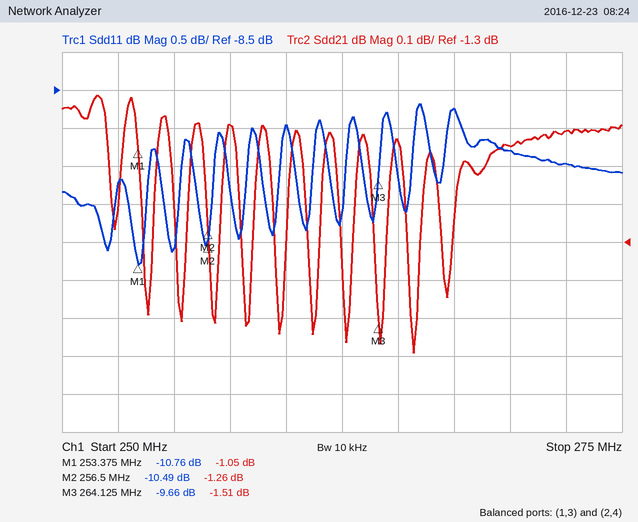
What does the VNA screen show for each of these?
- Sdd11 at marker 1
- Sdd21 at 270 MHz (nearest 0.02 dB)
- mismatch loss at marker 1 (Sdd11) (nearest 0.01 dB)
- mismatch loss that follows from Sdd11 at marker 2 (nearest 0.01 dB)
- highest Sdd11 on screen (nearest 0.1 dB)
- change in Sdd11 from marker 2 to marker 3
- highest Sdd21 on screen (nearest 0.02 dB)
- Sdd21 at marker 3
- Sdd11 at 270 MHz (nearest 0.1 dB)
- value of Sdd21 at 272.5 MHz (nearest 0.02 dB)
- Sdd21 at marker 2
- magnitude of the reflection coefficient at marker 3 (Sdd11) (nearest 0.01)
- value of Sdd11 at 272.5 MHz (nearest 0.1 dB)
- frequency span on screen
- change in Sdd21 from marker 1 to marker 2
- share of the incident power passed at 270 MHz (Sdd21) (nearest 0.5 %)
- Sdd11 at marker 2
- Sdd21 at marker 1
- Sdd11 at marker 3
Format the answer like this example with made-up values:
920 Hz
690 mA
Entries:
-10.76 dB
-1.04 dB
0.38 dB
0.41 dB
-8.7 dB
0.83 dB
-0.92 dB
-1.51 dB
-9.3 dB
-1.00 dB
-1.26 dB
0.33
-9.5 dB
25 MHz
-0.21 dB
78.5 %
-10.49 dB
-1.05 dB
-9.66 dB
